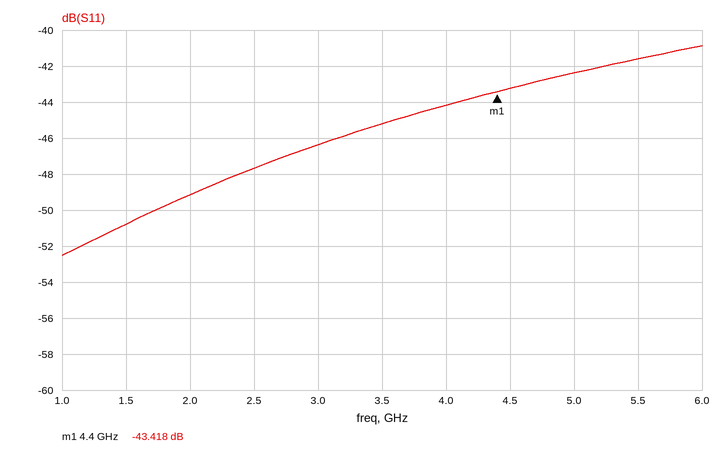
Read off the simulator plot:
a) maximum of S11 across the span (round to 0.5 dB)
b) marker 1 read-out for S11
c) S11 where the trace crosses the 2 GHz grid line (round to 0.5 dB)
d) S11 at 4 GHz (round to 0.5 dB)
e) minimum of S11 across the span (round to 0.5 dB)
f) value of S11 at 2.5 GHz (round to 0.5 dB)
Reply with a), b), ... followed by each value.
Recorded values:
a) -41.0 dB
b) -43.418 dB
c) -49.0 dB
d) -44.0 dB
e) -52.5 dB
f) -47.5 dB
